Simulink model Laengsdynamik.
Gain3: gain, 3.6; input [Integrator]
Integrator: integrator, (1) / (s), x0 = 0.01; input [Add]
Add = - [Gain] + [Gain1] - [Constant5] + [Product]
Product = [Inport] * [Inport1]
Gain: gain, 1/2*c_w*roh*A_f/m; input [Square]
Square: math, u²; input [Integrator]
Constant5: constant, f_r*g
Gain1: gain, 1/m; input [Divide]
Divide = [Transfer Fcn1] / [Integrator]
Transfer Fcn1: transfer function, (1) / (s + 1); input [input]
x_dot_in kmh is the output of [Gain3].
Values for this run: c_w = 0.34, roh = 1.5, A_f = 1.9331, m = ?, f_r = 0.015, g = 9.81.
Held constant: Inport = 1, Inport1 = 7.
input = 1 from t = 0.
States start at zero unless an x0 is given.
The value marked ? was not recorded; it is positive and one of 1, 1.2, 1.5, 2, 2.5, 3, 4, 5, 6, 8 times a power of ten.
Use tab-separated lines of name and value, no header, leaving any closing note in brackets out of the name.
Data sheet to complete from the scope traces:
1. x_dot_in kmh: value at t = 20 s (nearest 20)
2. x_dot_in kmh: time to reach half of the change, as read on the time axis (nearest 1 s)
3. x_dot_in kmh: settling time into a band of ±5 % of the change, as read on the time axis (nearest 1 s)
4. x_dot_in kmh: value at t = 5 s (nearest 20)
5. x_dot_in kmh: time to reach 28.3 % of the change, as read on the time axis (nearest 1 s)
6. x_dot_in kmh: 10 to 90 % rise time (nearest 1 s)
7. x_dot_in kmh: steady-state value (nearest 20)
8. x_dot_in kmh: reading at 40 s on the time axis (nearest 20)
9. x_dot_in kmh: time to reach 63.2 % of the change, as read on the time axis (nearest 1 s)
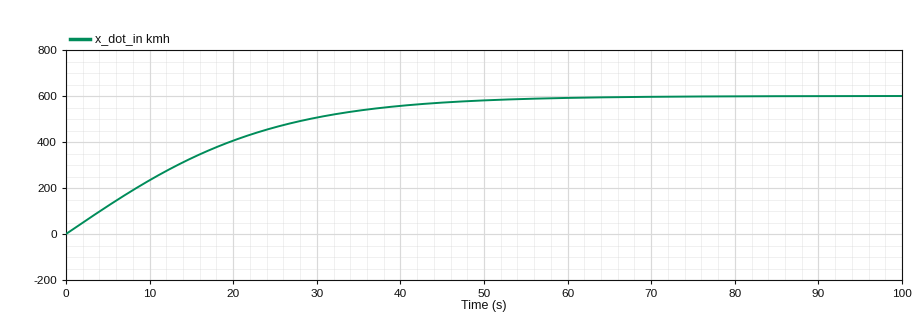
x_dot_in kmh: value at t = 20 s	400
x_dot_in kmh: time to reach half of the change, as read on the time axis	13 s
x_dot_in kmh: settling time into a band of ±5 % of the change, as read on the time axis	45 s
x_dot_in kmh: value at t = 5 s	120
x_dot_in kmh: time to reach 28.3 % of the change, as read on the time axis	7 s
x_dot_in kmh: 10 to 90 % rise time	33 s
x_dot_in kmh: steady-state value	600
x_dot_in kmh: reading at 40 s on the time axis	560
x_dot_in kmh: time to reach 63.2 % of the change, as read on the time axis	18 s
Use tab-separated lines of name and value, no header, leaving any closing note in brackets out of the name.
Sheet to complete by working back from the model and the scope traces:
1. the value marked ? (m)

the value marked ?	2000
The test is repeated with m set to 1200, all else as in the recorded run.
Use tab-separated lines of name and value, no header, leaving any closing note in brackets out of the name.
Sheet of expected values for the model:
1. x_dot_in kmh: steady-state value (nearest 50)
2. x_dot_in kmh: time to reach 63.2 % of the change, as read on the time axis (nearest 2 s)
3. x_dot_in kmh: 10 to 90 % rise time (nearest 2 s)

x_dot_in kmh: steady-state value	450
x_dot_in kmh: time to reach 63.2 % of the change, as read on the time axis	14 s
x_dot_in kmh: 10 to 90 % rise time	26 s
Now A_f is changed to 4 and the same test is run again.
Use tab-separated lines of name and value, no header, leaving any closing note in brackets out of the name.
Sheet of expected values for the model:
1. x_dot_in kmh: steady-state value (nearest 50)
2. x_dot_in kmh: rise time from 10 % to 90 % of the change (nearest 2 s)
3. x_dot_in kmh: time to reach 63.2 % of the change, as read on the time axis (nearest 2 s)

x_dot_in kmh: steady-state value	400
x_dot_in kmh: rise time from 10 % to 90 % of the change	24 s
x_dot_in kmh: time to reach 63.2 % of the change, as read on the time axis	12 s
